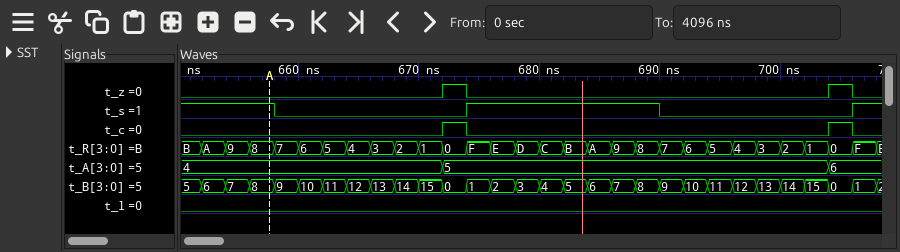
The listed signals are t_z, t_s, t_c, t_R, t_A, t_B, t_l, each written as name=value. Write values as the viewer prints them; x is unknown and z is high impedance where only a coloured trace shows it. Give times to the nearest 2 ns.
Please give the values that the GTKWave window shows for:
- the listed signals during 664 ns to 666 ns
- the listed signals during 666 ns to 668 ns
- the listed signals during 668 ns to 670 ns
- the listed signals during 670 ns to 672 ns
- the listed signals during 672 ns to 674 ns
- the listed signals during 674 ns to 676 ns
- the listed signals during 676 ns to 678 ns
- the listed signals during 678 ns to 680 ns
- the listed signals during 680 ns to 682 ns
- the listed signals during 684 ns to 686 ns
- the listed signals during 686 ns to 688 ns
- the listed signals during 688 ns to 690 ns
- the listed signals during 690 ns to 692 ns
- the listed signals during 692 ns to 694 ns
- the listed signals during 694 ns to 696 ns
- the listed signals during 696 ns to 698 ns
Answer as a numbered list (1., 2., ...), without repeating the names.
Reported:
1. t_z=0, t_s=0, t_c=0, t_R=4, t_A=4, t_B=12, t_l=0
2. t_z=0, t_s=0, t_c=0, t_R=3, t_A=4, t_B=13, t_l=0
3. t_z=0, t_s=0, t_c=0, t_R=2, t_A=4, t_B=14, t_l=0
4. t_z=0, t_s=0, t_c=0, t_R=1, t_A=4, t_B=15, t_l=0
5. t_z=1, t_s=0, t_c=1, t_R=0, t_A=5, t_B=0, t_l=0
6. t_z=0, t_s=1, t_c=0, t_R=F, t_A=5, t_B=1, t_l=0
7. t_z=0, t_s=1, t_c=0, t_R=E, t_A=5, t_B=2, t_l=0
8. t_z=0, t_s=1, t_c=0, t_R=D, t_A=5, t_B=3, t_l=0
9. t_z=0, t_s=1, t_c=0, t_R=C, t_A=5, t_B=4, t_l=0
10. t_z=0, t_s=1, t_c=0, t_R=A, t_A=5, t_B=6, t_l=0
11. t_z=0, t_s=1, t_c=0, t_R=9, t_A=5, t_B=7, t_l=0
12. t_z=0, t_s=1, t_c=0, t_R=8, t_A=5, t_B=8, t_l=0
13. t_z=0, t_s=0, t_c=0, t_R=7, t_A=5, t_B=9, t_l=0
14. t_z=0, t_s=0, t_c=0, t_R=6, t_A=5, t_B=10, t_l=0
15. t_z=0, t_s=0, t_c=0, t_R=5, t_A=5, t_B=11, t_l=0
16. t_z=0, t_s=0, t_c=0, t_R=4, t_A=5, t_B=12, t_l=0
